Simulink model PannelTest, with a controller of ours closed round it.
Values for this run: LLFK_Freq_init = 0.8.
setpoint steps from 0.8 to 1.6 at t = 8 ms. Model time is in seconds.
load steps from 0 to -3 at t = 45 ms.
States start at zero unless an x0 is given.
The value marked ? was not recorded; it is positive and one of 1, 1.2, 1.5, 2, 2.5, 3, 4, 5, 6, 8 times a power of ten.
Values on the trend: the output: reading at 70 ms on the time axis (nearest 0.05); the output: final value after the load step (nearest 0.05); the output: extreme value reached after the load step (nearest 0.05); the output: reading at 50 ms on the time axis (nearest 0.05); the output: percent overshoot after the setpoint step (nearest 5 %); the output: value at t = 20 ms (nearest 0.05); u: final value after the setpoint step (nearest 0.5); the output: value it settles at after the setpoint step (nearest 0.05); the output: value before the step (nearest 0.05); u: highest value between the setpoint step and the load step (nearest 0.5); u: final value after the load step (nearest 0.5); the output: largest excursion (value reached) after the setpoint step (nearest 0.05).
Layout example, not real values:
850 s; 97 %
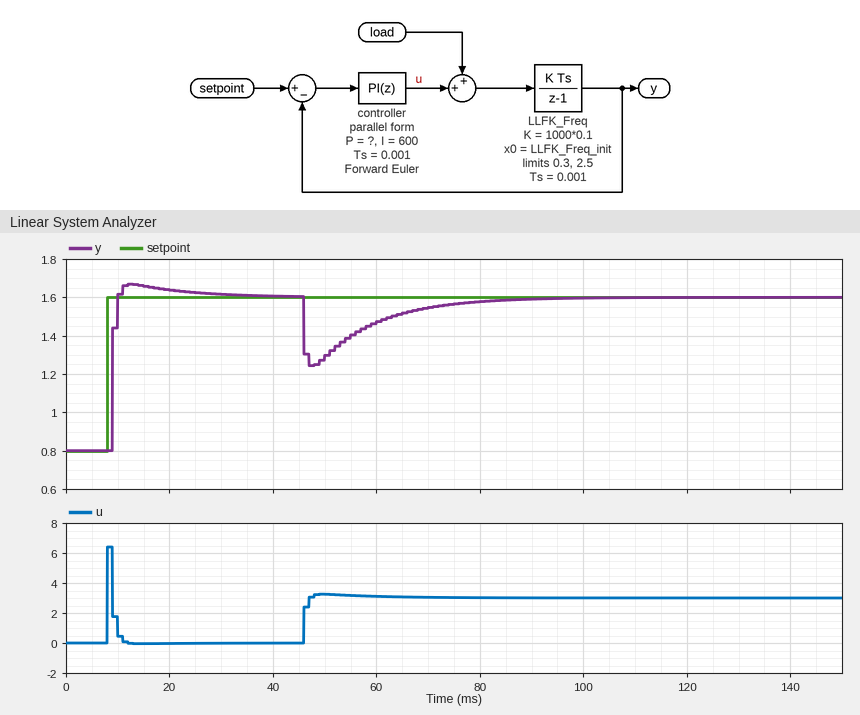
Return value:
1.55; 1.60; 1.25; 1.30; 10 %; 1.65; 0.0; 1.60; 0.80; 6.5; 3.0; 1.65
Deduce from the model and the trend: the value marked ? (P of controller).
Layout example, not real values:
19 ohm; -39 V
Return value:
8
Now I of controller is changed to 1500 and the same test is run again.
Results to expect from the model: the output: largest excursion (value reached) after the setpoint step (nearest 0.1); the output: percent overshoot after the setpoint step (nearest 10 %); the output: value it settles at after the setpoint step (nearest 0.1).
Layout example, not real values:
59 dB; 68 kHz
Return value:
1.8; 20 %; 1.6
